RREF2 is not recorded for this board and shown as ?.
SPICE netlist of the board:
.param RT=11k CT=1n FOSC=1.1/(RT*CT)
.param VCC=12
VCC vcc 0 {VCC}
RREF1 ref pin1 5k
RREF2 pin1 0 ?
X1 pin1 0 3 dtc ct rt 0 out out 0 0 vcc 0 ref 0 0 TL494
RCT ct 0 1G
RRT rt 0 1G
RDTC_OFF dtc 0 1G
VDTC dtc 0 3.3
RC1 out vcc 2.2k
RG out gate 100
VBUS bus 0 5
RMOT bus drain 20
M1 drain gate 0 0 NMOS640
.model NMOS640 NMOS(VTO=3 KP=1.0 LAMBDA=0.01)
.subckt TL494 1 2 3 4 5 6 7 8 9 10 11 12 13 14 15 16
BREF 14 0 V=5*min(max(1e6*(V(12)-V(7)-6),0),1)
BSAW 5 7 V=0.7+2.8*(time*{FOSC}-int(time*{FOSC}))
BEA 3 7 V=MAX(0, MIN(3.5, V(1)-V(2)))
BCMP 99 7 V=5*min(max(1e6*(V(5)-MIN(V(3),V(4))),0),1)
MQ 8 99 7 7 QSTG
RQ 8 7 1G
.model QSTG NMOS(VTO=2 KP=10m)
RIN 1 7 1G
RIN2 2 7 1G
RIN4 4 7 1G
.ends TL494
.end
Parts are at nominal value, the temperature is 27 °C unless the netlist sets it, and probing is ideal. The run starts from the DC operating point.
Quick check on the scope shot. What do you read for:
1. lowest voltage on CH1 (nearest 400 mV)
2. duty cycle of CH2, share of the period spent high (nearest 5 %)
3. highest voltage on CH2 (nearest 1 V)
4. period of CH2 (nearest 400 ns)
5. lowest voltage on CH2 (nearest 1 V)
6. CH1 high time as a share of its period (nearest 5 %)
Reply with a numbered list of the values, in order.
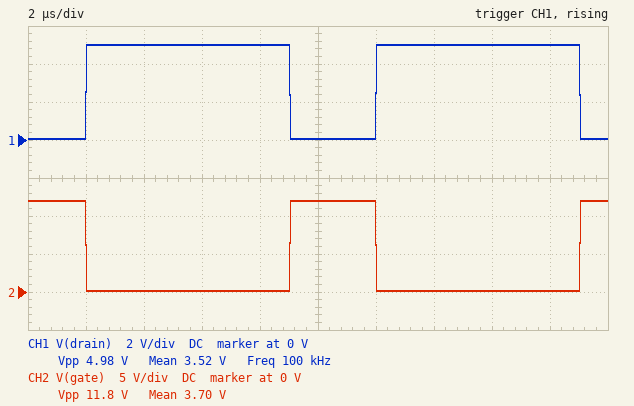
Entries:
1. 0 V
2. 30 %
3. 12 V
4. 10.0 µs
5. 0 V
6. 70 %
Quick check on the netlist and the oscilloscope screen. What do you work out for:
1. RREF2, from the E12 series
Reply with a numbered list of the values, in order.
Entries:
1. 2.2 kΩ
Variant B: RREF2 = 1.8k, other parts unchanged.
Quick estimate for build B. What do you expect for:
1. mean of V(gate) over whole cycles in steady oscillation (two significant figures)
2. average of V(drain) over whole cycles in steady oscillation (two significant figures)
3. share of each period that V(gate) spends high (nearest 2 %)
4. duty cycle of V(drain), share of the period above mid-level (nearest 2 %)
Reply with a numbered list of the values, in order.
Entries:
1. 2.8 V
2. 3.9 V
3. 22 %
4. 78 %
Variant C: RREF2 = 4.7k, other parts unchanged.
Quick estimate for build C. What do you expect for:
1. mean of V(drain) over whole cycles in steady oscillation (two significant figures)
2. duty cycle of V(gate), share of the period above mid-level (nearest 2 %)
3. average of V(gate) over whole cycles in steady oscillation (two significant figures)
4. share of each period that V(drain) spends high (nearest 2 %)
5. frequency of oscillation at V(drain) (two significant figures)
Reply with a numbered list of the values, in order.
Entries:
1. 1.9 V
2. 62 %
3. 7.5 V
4. 38 %
5. 100 kHz
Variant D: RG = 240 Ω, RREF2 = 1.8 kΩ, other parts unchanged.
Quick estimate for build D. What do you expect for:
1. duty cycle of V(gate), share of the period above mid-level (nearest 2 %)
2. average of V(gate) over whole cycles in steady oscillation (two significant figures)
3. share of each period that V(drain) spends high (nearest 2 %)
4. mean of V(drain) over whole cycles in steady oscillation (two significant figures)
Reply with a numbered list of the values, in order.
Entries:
1. 22 %
2. 2.8 V
3. 78 %
4. 3.9 V
